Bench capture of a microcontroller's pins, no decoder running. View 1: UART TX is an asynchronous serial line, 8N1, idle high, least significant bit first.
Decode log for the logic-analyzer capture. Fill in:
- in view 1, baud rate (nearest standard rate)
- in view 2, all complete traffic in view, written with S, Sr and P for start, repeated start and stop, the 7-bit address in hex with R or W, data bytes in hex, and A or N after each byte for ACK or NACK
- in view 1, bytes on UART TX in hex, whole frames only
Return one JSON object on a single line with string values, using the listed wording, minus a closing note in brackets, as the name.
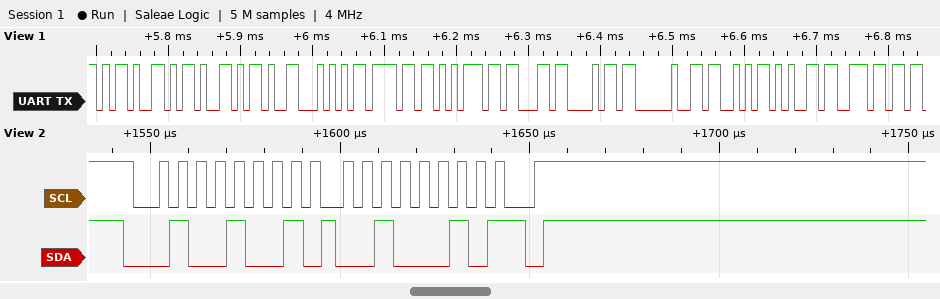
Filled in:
{"in view 1, baud rate": "115200 baud", "in view 2, all complete traffic in view, written with S, Sr and P for start, repeated start and stop, the 7-bit address in hex with R or W, data bytes in hex, and A or N after each byte for ACK or NACK": "S 24R A 22 N P", "in view 1, bytes on UART TX in hex, whole frames only": "2D 2D 2D 54 6F 75 63 68 20 53 65 6E"}
